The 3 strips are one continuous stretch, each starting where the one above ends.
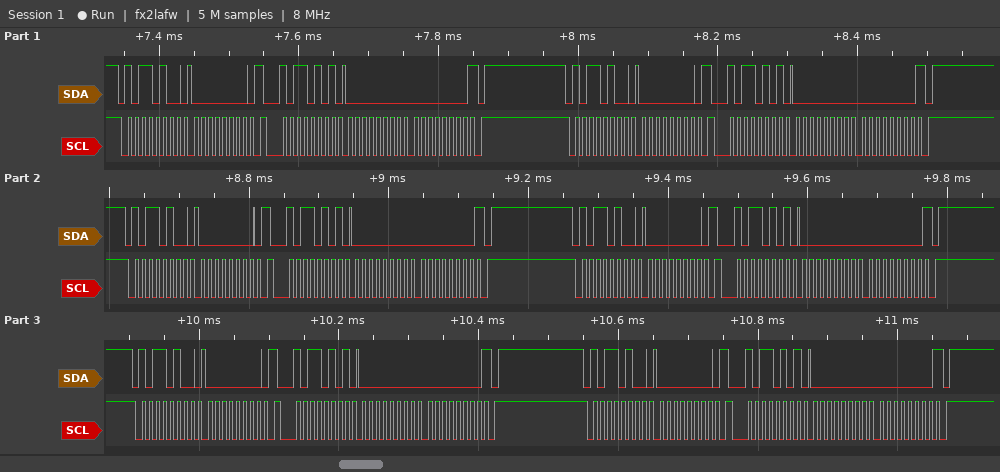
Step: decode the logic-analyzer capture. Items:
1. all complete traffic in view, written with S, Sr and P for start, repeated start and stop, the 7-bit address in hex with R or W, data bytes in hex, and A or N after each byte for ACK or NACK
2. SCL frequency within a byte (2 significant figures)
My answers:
S 5AW A 00 A Sr 5AR A 00 A 00 N P S 5AW A 00 A Sr 5AR A 00 A 00 N P S 5AW A 00 A Sr 5AR A 00 A 00 N P S 5AW A 00 A Sr 5AR A 00 A 00 N P S 5AW A 00 A Sr 5AR A 00 A 00 N P S 5AW A 00 A Sr 5AR A 00 A 00 N P
100 kHz
